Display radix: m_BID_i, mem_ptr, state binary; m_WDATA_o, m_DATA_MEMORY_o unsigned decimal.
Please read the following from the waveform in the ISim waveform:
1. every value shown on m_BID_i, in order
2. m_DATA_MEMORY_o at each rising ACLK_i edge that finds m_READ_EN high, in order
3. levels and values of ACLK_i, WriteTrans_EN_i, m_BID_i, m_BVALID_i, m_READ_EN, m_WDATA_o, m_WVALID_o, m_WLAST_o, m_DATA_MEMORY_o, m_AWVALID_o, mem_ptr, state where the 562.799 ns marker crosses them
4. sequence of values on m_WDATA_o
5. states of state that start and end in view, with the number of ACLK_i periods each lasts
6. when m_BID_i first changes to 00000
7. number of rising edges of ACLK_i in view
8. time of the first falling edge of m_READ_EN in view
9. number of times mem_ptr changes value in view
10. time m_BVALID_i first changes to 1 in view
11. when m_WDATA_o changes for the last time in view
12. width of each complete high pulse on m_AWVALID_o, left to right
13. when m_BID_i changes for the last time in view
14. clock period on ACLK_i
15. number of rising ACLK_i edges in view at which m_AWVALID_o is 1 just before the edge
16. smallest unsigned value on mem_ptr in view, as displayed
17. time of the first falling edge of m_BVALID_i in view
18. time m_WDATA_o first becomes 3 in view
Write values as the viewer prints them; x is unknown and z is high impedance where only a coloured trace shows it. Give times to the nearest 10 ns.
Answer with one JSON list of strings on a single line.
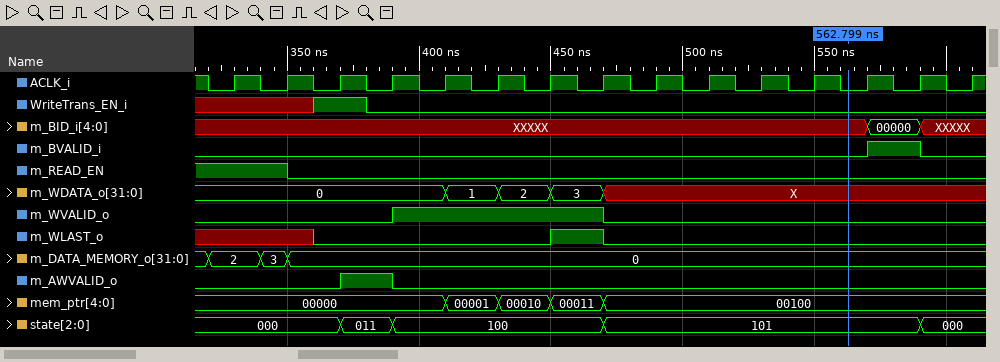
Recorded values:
["XXXXX, 00000, XXXXX", "2, 3", "ACLK_i=0, WriteTrans_EN_i=0, m_BID_i=XXXXX, m_BVALID_i=0, m_READ_EN=0, m_WDATA_o=X, m_WVALID_o=0, m_WLAST_o=0, m_DATA_MEMORY_o=0, m_AWVALID_o=0, mem_ptr=00100, state=101", "0, 1, 2, 3, X", "011: 1, 100: 4, 101: 6", "570 ns", "15", "350 ns", "4", "570 ns", "470 ns", "20 ns", "590 ns", "20 ns", "1", "00000", "590 ns", "450 ns"]
